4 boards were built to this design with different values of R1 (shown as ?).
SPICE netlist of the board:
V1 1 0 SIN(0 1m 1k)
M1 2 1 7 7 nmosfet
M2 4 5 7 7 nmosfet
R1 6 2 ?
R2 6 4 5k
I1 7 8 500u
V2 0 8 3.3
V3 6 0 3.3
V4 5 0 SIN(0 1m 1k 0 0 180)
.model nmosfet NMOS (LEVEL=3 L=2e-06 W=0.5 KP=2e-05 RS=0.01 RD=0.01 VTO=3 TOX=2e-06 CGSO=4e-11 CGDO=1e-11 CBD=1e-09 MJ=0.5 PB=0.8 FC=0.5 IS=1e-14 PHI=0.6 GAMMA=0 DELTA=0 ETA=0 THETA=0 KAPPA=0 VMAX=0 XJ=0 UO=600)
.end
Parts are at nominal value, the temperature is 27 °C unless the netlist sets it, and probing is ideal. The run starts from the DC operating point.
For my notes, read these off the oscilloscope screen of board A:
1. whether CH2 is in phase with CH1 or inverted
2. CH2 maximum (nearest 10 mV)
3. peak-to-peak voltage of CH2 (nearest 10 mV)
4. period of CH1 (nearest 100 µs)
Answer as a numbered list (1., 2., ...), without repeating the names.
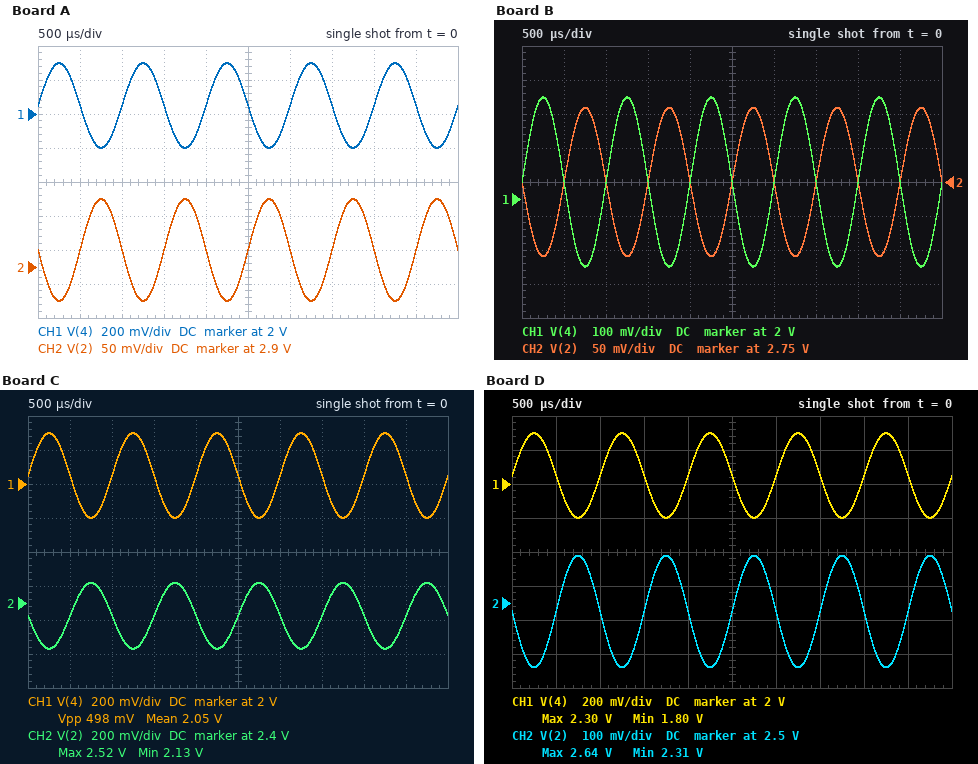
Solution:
1. inverted
2. 3.00 V
3. 150 mV
4. 1.0 ms
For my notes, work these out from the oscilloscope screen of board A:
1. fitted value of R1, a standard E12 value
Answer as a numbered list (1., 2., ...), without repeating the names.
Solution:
1. 1.5 kΩ
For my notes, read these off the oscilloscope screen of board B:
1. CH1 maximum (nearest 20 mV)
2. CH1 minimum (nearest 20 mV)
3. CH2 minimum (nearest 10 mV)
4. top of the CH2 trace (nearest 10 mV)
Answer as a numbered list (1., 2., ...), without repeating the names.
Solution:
1. 2.30 V
2. 1.80 V
3. 2.64 V
4. 2.86 V
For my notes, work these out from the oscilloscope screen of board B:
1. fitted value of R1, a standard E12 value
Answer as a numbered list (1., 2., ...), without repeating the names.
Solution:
1. 2.2 kΩ
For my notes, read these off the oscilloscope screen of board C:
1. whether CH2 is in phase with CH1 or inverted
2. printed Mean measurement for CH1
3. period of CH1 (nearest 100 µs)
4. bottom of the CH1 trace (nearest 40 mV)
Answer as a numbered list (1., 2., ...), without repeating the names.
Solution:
1. inverted
2. 2.05 V
3. 1.0 ms
4. 1.80 V
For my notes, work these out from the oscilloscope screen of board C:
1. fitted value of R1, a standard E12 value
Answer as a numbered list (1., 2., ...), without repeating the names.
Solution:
1. 3.9 kΩ
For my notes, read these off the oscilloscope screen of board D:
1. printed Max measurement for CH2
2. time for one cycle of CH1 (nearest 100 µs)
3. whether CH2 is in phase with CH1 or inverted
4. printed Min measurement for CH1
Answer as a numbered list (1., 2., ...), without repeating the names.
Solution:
1. 2.64 V
2. 1.0 ms
3. inverted
4. 1.80 V
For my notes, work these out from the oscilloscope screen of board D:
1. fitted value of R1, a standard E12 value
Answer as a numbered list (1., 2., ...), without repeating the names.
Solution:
1. 3.3 kΩ
